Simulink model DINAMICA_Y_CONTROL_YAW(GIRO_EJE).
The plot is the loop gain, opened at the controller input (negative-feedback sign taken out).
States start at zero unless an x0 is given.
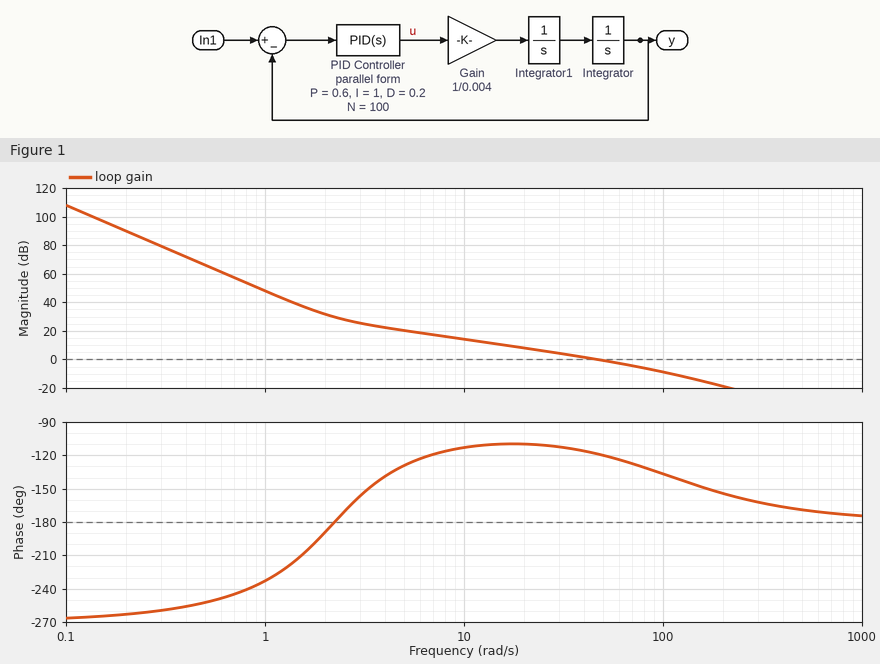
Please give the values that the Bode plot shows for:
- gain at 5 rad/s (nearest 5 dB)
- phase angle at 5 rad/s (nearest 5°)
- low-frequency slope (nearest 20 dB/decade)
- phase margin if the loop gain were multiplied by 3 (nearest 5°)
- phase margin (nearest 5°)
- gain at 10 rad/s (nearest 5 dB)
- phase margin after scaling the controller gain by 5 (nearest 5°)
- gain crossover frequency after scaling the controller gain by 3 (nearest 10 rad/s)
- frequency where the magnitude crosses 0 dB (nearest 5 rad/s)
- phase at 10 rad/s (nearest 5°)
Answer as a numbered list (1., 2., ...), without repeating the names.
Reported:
1. 20 dB
2. -130°
3. -60 dB/decade
4. 40°
5. 60°
6. 15 dB
7. 35°
8. 110 rad/s
9. 45 rad/s
10. -115°
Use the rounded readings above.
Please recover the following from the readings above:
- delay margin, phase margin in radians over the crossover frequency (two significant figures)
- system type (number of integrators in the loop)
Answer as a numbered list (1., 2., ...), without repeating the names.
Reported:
1. 0.023 s
2. 3
